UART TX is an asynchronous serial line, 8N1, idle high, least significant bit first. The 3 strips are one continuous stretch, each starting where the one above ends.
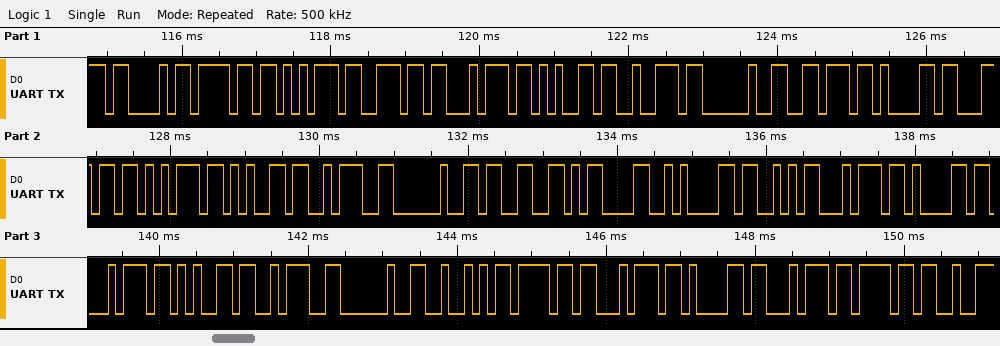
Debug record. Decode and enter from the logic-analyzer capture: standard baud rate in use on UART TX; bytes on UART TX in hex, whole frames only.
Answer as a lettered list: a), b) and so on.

a) 9600 baud
b) 43 6F 75 6E 74 65 72 20 76 61 6C 75 65 3A 20 33 0D 0A 53 74 61 74 65 3A 20 52 6F 74 61 74 6F
